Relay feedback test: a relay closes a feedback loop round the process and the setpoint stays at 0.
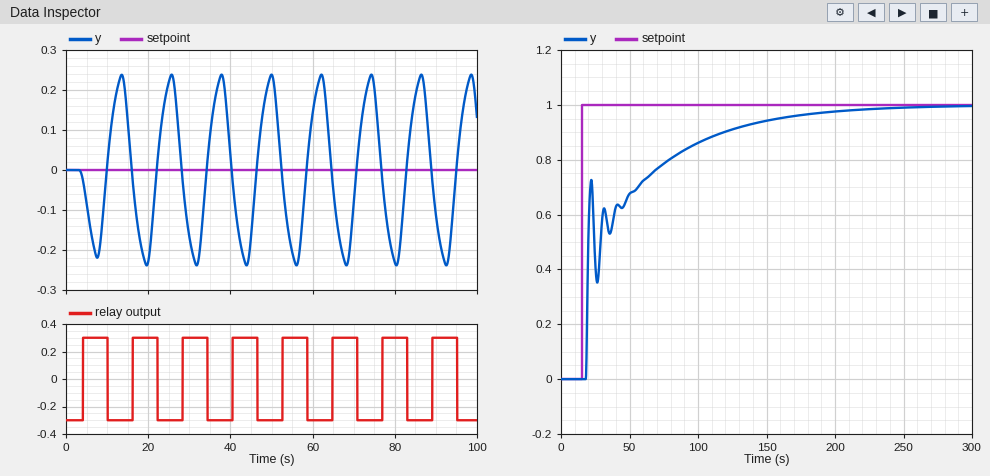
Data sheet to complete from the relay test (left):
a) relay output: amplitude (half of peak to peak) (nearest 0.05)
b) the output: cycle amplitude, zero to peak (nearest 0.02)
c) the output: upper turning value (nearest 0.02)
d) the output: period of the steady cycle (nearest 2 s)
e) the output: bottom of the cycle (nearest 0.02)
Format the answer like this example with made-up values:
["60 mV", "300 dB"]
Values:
["0.30", "0.24", "0.24", "12 s", "-0.24"]
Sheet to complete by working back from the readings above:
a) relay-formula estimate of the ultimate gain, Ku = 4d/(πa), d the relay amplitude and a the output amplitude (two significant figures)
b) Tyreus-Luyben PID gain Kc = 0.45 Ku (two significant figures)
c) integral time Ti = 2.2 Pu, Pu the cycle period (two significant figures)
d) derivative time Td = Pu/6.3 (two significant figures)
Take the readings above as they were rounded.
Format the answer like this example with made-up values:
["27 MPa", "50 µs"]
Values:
["1.6", "0.72", "26 s", "1.9 s"]
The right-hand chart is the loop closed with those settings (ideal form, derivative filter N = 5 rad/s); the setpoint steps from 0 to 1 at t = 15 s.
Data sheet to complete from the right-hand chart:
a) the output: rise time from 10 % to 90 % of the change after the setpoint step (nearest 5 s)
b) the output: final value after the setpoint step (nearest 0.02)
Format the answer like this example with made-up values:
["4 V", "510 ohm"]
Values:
["100 s", "1.00"]
